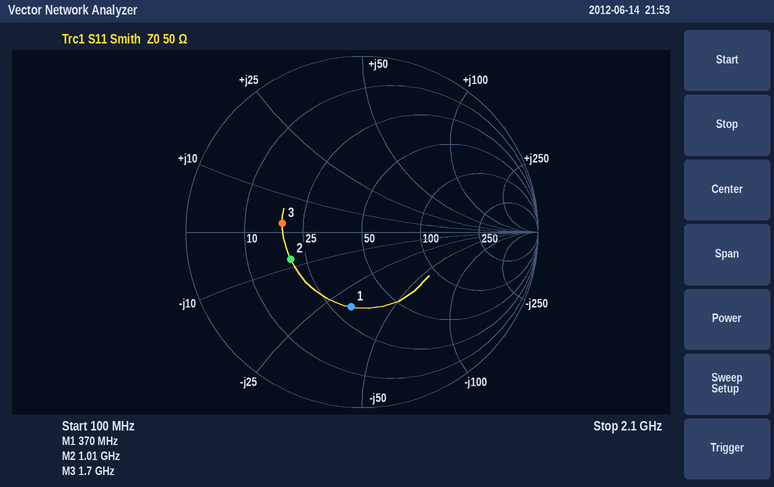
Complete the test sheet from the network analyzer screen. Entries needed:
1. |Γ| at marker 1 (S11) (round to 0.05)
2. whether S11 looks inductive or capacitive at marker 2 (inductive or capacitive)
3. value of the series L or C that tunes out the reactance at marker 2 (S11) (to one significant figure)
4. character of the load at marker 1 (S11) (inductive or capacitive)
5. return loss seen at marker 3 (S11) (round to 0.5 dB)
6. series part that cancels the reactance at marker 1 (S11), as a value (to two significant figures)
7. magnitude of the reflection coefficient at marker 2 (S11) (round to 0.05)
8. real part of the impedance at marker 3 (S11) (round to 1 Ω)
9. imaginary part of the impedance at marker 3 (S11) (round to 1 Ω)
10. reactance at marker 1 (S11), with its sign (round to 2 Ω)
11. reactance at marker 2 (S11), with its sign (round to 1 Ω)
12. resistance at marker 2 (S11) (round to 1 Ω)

0.45
capacitive
1 nH
capacitive
7.0 dB
14 nH
0.45
19 Ω
+2 Ω
-32 Ω
-8 Ω
20 Ω
